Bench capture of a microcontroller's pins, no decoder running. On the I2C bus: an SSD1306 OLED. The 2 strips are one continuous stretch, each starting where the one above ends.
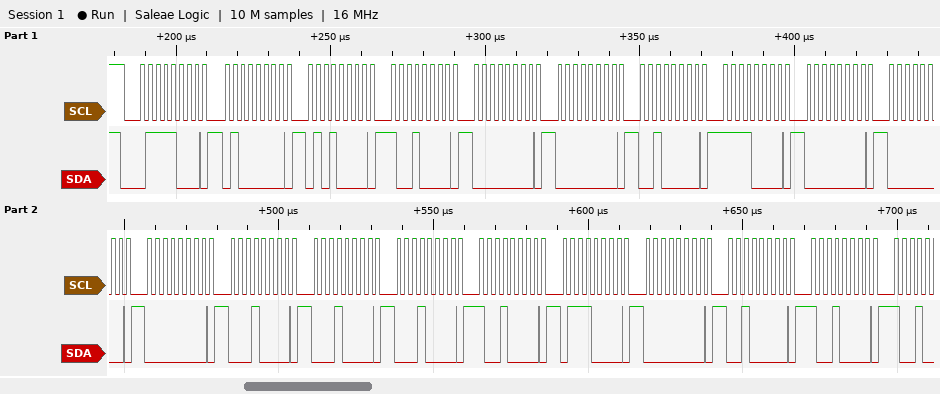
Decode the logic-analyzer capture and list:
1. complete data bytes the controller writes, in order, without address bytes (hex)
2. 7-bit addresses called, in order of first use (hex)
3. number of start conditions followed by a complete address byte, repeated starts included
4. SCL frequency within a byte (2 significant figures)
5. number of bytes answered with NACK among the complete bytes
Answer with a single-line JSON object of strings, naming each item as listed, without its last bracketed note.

{"complete data bytes the controller writes, in order, without address bytes": "40 50 90 00 00 20 F0 00 00 00 10 10 10 90 70 00 20 90", "7-bit addresses called, in order of first use": "0x3C", "number of start conditions followed by a complete address byte, repeated starts included": "1", "SCL frequency within a byte": "400 kHz", "number of bytes answered with NACK among the complete bytes": "0"}
